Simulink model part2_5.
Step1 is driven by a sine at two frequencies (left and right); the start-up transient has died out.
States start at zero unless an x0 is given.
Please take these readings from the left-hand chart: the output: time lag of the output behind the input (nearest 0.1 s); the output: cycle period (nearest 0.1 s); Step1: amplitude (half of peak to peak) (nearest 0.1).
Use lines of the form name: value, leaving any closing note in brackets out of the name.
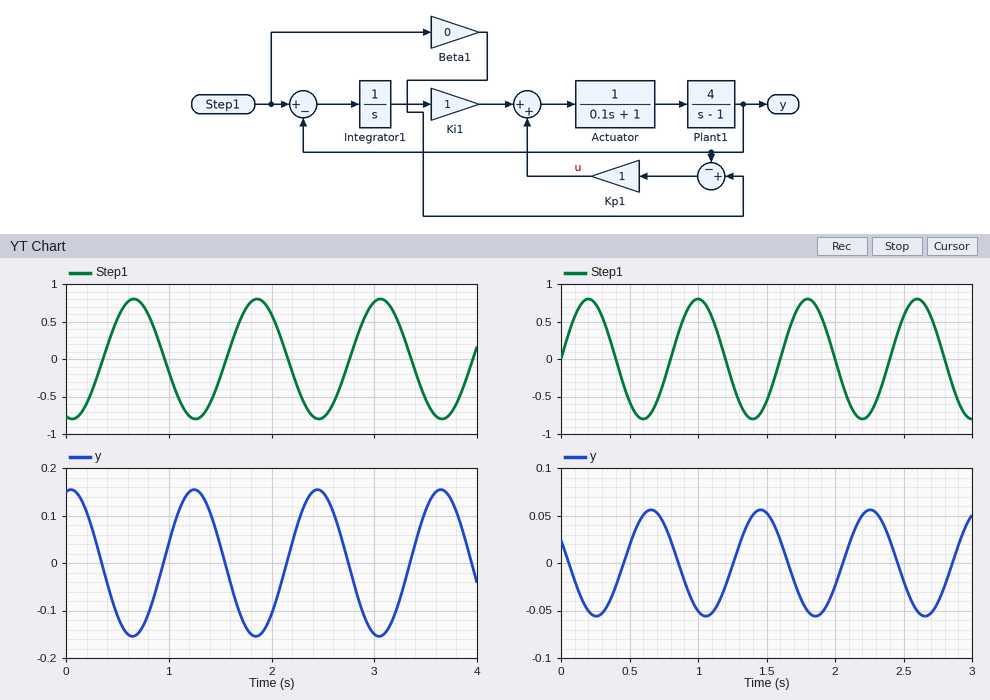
the output: time lag of the output behind the input: 0.6 s
the output: cycle period: 1.2 s
Step1: amplitude (half of peak to peak): 0.8
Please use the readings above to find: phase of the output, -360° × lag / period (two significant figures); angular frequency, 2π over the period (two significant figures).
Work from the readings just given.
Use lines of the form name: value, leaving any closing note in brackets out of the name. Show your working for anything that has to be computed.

phase of the output, -360° × lag / period: -360 × 0.6 / 1.2 = -180°
angular frequency, 2π over the period: 2π / 1.2 = 5.2 rad/s
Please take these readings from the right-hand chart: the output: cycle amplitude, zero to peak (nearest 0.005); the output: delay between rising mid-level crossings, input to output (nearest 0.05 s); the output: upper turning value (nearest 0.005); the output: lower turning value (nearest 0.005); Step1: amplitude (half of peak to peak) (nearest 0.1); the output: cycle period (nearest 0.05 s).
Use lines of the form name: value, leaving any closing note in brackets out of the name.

the output: cycle amplitude, zero to peak: 0.055
the output: delay between rising mid-level crossings, input to output: 0.45 s
the output: upper turning value: 0.055
the output: lower turning value: -0.055
Step1: amplitude (half of peak to peak): 0.8
the output: cycle period: 0.80 s
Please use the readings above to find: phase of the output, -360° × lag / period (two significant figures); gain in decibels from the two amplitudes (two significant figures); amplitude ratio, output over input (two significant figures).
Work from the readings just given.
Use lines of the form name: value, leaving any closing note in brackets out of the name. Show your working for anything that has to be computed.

phase of the output, -360° × lag / period: -360 × 0.45 / 0.8 = -200°
gain in decibels from the two amplitudes: 20 log10(0.055 / 0.8) = -23 dB
amplitude ratio, output over input: 0.055 / 0.8 = 0.069
